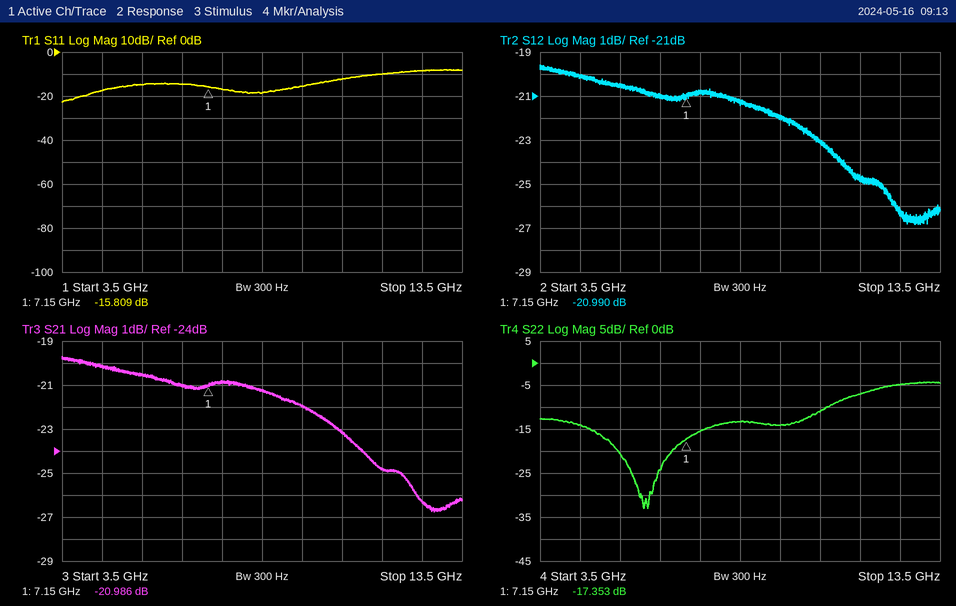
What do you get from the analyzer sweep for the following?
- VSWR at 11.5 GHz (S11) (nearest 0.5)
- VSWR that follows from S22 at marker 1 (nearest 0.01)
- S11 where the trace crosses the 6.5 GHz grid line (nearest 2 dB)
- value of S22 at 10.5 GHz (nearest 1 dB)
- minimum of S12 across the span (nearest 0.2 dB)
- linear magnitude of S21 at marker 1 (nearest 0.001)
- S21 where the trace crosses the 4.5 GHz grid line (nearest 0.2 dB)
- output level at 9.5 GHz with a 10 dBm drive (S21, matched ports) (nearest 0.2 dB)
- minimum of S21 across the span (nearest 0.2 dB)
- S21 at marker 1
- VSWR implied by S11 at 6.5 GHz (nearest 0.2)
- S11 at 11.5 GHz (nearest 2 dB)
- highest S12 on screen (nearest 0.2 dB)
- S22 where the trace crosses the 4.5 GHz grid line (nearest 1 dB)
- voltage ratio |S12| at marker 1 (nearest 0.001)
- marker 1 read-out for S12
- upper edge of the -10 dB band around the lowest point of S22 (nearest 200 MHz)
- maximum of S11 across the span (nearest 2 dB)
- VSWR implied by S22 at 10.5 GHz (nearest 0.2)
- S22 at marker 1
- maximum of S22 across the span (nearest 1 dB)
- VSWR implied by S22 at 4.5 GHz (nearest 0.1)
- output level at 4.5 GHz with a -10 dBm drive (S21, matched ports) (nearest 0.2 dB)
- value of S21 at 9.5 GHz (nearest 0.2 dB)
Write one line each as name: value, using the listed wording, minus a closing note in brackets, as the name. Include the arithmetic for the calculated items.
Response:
VSWR at 11.5 GHz (S11): |Γ| = 10^(-10/20) = 0.3162; VSWR = (1 + 0.3162)/(1 − 0.3162) ≈ 1.92, so 2.0 to the nearest 0.5
VSWR that follows from S22 at marker 1: (1 + 0.1356)/(1 − 0.1356) ≈ 1.31
S11 where the trace crosses the 6.5 GHz grid line: -14 dB
value of S22 at 10.5 GHz: -11 dB
minimum of S12 across the span: -26.8 dB
linear magnitude of S21 at marker 1: 10^(-20.986/20) ≈ 0.089
S21 where the trace crosses the 4.5 GHz grid line: -20.2 dB
output level at 9.5 GHz with a 10 dBm drive (S21, matched ports): 10 dBm + (-22.0 dB) = -12.0 dBm
minimum of S21 across the span: -26.8 dB
S21 at marker 1: -20.986 dB
VSWR implied by S11 at 6.5 GHz: |Γ| = 10^(-14/20) = 0.1995; VSWR = (1 + 0.1995)/(1 − 0.1995) ≈ 1.50, so 1.4 to the nearest 0.2
S11 at 11.5 GHz: -10 dB
highest S12 on screen: -19.6 dB
S22 where the trace crosses the 4.5 GHz grid line: -14 dB
voltage ratio |S12| at marker 1: 10^(-20.99/20) ≈ 0.089
marker 1 read-out for S12: -20.990 dB
upper edge of the -10 dB band around the lowest point of S22: 10.6 GHz
maximum of S11 across the span: -8 dB
VSWR implied by S22 at 10.5 GHz: |Γ| = 10^(-11/20) = 0.2818; VSWR = (1 + 0.2818)/(1 − 0.2818) ≈ 1.8
S22 at marker 1: -17.353 dB
maximum of S22 across the span: -4 dB
VSWR implied by S22 at 4.5 GHz: |Γ| = 10^(-14/20) = 0.1995; VSWR = (1 + 0.1995)/(1 − 0.1995) ≈ 1.5
output level at 4.5 GHz with a -10 dBm drive (S21, matched ports): -10 dBm + (-20.2 dB) = -30.2 dBm
value of S21 at 9.5 GHz: -22.0 dB
